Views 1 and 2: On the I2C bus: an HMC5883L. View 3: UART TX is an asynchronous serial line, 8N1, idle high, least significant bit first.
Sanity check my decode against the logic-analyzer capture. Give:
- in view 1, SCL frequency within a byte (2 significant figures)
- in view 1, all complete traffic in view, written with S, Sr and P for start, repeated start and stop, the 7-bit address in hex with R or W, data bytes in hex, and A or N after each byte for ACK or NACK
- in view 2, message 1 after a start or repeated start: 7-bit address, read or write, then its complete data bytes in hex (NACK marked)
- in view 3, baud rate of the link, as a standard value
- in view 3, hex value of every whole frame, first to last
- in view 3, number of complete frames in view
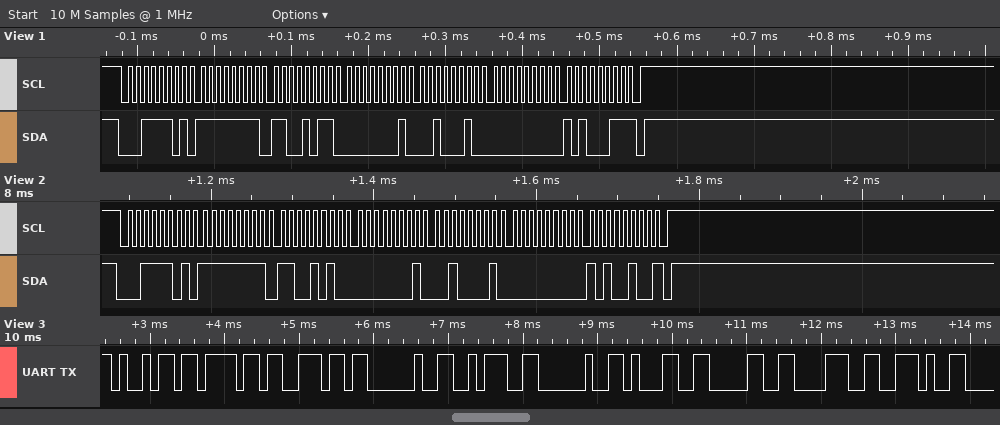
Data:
100 kHz
S 1ER A FF A CB A 01 A 22 A 00 A A3 N P
0x1E read: FF CA 01 21 00 A4 NACK
9600 baud
69 6F 6E 20 3A 20 31 30 38 2E
10
